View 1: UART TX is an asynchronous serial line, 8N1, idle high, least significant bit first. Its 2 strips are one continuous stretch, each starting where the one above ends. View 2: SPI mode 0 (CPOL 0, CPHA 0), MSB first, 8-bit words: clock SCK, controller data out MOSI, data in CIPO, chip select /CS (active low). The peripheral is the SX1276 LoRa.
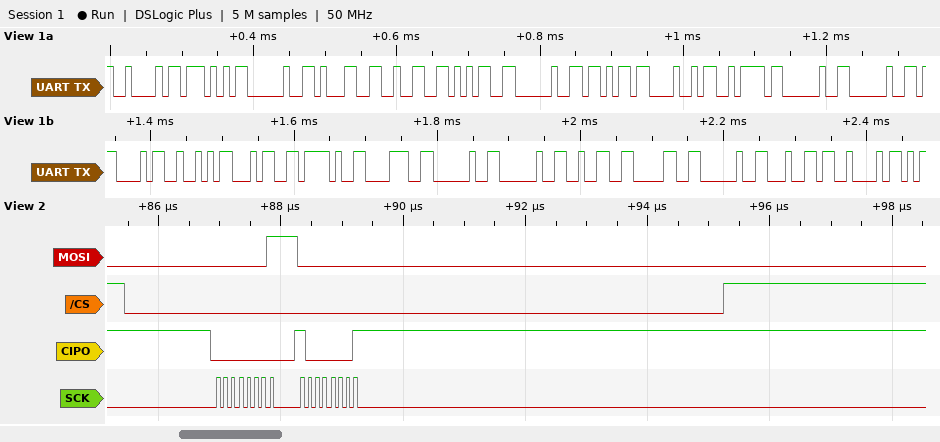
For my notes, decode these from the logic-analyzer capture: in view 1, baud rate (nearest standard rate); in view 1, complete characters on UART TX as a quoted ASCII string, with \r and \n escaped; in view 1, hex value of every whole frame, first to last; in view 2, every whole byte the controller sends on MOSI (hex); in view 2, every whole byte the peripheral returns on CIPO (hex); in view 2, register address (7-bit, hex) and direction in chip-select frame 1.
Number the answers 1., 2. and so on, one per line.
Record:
1. 115200 baud
2. "BW 125 kHz  CR4/8  20 dB"
3. 42 57 20 31 32 35 20 6B 48 7A 20 20 43 52 34 2F 38 20 20 32 30 20 64 42
4. 01 00
5. 00 81
6. 0x01 read
